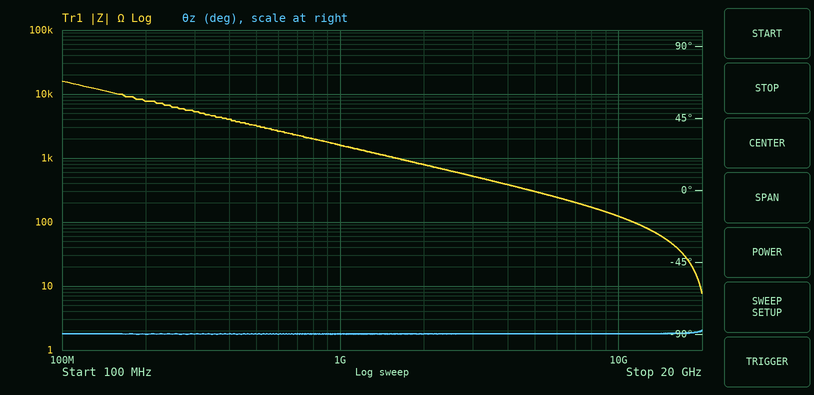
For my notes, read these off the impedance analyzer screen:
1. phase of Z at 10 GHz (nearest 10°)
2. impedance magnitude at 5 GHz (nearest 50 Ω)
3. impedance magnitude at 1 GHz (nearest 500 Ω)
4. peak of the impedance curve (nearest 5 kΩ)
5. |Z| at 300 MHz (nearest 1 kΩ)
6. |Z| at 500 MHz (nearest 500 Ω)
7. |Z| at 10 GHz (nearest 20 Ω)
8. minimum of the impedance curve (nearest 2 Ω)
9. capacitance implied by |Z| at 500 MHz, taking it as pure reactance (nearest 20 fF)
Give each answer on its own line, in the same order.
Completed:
-90°
300 Ω
1.5 kΩ
15 kΩ
5 kΩ
3.0 kΩ
120 Ω
8 Ω
100 fF
